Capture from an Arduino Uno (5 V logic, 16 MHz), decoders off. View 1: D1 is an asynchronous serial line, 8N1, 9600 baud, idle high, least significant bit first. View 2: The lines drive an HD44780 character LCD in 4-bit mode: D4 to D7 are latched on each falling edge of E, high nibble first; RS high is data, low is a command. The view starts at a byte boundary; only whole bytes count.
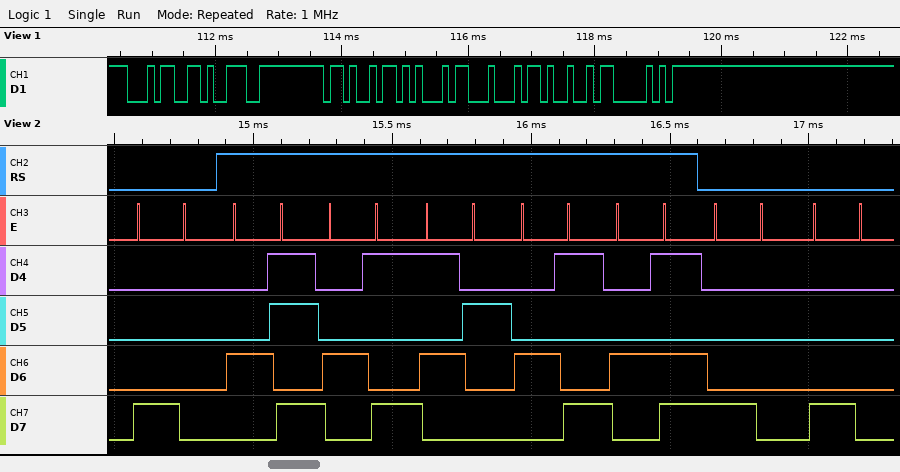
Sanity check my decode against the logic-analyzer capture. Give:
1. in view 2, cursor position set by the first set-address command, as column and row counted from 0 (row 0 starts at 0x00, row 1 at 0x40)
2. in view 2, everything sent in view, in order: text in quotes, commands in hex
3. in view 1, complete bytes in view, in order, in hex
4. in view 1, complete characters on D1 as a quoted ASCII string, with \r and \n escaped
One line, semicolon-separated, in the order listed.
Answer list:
column 0, row 0; 0x80 "KIRIM" 0x80 0x80; 34 39 4B 45 44 49 50; "49KEDIP"
